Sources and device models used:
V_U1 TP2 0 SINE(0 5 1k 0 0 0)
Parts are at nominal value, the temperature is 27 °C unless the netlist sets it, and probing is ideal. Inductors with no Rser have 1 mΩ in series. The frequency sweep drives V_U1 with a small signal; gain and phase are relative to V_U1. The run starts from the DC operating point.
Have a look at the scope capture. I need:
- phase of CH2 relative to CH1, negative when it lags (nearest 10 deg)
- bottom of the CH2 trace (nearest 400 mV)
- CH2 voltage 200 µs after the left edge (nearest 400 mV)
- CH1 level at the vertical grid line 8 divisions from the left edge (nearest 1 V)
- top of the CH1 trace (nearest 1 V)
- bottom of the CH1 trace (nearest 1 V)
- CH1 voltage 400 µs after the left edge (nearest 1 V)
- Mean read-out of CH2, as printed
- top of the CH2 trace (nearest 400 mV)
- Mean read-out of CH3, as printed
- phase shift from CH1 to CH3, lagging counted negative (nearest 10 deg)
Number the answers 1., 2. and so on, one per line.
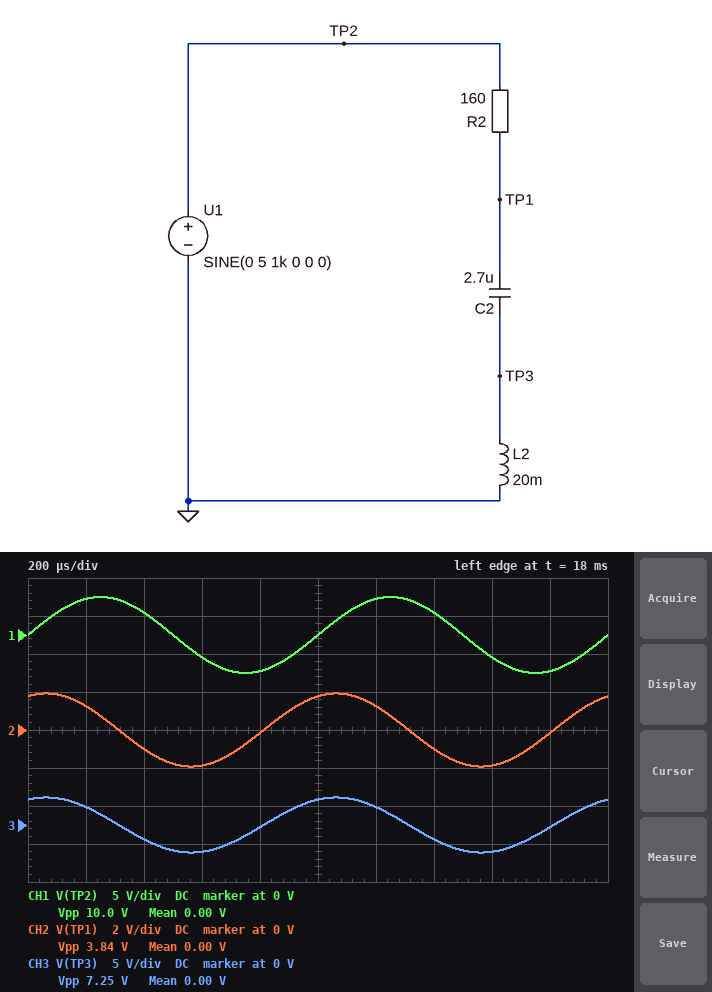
1. 70 deg
2. -2.0 V
3. 1.2 V
4. -3 V
5. 5 V
6. -5 V
7. 3 V
8. 0.00 V
9. 2.0 V
10. 0.00 V
11. 70 deg
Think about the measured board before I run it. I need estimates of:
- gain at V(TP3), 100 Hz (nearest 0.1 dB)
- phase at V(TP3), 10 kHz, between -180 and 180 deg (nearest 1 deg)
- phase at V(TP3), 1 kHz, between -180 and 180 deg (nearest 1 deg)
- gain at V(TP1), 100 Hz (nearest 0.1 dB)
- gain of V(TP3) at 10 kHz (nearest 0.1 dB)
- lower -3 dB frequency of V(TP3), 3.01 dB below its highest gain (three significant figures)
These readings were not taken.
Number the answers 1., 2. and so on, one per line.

1. -33.6 dB
2. 7 deg
3. 67 deg
4. -0.3 dB
5. 0 dB
6. 960 Hz
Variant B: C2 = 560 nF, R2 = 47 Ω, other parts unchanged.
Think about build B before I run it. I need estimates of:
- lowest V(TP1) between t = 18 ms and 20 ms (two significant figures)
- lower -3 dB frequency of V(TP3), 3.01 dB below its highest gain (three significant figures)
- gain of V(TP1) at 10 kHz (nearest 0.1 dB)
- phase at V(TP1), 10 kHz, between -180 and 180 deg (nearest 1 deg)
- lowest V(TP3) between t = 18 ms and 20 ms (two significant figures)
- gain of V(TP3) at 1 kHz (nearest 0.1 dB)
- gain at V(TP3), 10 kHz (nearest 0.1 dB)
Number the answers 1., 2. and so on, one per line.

1. -4.8 V
2. 1.36 kHz
3. 0 dB
4. 2 deg
5. -3.8 V
6. -2.4 dB
7. 0.2 dB
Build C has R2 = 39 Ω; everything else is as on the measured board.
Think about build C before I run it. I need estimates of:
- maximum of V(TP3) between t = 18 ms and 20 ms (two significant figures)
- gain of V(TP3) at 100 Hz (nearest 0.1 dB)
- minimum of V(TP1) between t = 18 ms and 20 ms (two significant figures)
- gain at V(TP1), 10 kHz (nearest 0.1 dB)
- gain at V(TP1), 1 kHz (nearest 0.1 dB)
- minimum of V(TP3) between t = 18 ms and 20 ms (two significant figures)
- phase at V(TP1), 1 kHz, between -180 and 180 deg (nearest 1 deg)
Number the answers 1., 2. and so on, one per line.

1. 8.1 V
2. -33.3 dB
3. -4.3 V
4. 0 dB
5. -1.3 dB
6. -8.1 V
7. 30 deg
